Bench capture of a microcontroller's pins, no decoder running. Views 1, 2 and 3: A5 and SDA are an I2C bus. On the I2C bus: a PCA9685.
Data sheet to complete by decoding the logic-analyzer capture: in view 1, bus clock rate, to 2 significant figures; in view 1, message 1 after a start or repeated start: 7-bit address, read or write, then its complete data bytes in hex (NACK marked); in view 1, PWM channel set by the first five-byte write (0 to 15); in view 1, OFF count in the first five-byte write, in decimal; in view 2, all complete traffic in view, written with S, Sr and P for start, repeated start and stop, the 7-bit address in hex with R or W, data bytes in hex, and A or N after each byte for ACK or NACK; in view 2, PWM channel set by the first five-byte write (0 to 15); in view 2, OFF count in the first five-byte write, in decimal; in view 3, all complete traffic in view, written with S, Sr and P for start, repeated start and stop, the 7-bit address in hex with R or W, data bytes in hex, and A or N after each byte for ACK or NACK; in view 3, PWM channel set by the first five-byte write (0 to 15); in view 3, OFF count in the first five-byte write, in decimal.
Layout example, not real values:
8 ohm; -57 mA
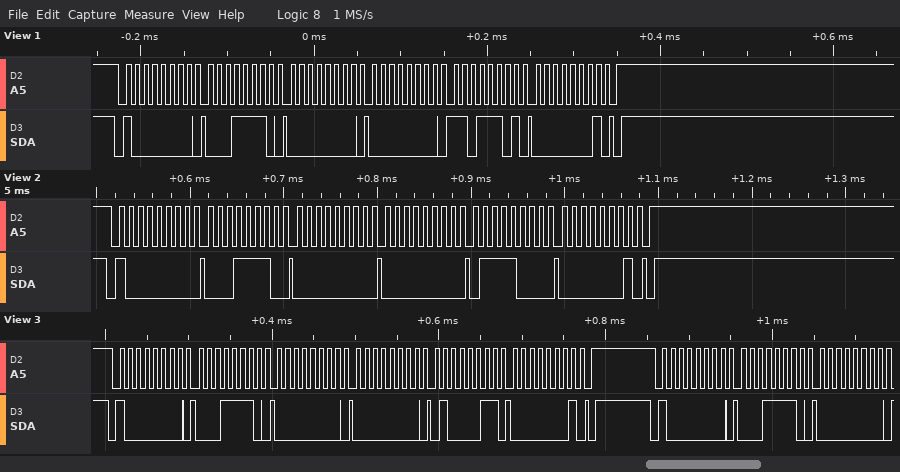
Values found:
100 kHz; 0x40 write: 1E 00 00 DD 01; 6; 477; S 40W A 1E A 00 A 00 A 78 A 01 A P; 6; 376; S 40W A 1E A 00 A 00 A 43 A 01 A P S 40W A 1E A 00 A; 6; 323
